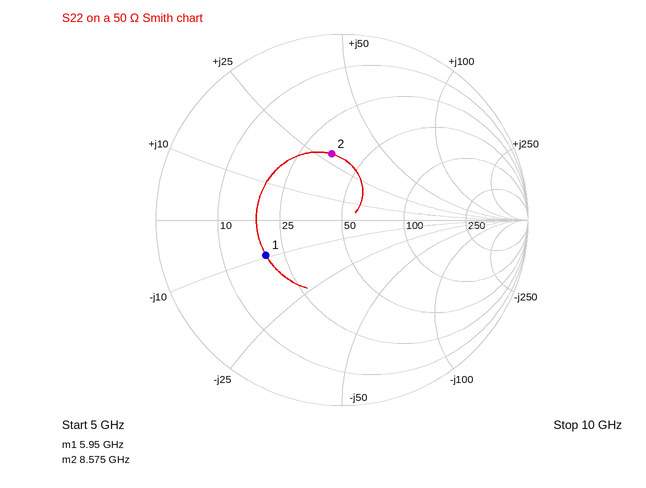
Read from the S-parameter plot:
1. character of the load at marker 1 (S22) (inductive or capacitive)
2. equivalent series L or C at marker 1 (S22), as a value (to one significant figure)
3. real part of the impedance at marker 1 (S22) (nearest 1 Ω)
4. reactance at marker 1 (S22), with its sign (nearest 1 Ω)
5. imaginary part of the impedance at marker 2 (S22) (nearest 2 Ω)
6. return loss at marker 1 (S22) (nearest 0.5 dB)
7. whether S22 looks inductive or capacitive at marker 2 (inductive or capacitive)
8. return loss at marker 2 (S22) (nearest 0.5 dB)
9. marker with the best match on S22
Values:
capacitive
3 pF
20 Ω
-9 Ω
+28 Ω
7.0 dB
inductive
9.0 dB
marker 2
